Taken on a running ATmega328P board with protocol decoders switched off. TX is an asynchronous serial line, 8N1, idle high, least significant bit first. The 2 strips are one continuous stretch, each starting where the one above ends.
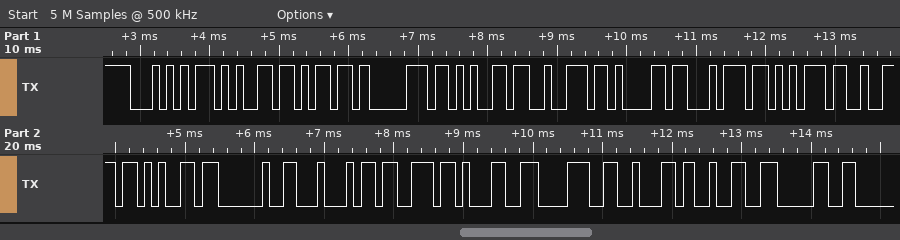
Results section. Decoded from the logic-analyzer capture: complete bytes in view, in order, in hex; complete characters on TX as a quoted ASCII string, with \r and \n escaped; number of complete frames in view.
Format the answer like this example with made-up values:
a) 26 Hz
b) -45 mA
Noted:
a) 0x54 0x65 0x6D 0x70 0x65 0x72 0x61 0x74 0x75 0x72 0x65 0x20 0x44 0x73 0x31 0x38 0x62 0x32 0x30
b) "Temperature Ds18b20"
c) 19
